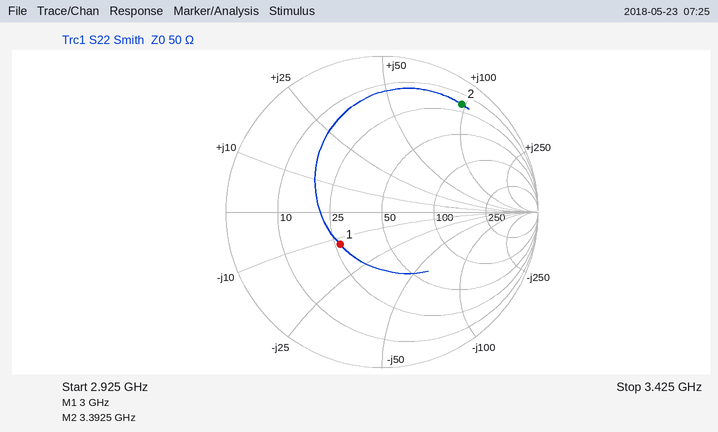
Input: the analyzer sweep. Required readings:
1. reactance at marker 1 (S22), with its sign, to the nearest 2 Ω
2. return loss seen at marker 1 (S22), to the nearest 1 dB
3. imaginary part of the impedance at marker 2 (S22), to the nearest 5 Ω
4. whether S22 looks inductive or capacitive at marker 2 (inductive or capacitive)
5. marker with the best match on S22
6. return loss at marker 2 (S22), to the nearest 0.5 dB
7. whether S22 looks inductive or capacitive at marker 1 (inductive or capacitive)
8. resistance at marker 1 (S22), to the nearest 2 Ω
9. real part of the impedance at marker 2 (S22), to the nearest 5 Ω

-12 Ω
9 dB
+95 Ω
inductive
marker 1
1.5 dB
capacitive
26 Ω
20 Ω
